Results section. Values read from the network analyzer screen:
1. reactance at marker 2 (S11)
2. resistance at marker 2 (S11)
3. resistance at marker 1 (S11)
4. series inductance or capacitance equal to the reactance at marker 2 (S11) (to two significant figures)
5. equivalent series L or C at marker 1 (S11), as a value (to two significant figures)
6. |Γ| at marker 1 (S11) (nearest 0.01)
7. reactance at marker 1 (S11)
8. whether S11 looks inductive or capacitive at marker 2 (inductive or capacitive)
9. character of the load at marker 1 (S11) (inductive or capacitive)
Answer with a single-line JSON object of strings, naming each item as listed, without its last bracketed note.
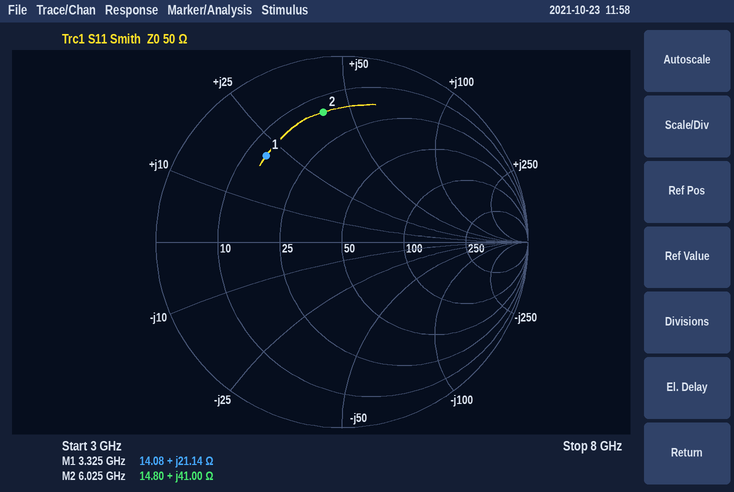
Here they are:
{"reactance at marker 2": "+41.00 Ω", "resistance at marker 2": "14.80 Ω", "resistance at marker 1": "14.08 Ω", "series inductance or capacitance equal to the reactance at marker 2 (S11)": "1.1 nH", "equivalent series L or C at marker 1 (S11), as a value": "1.0 nH", "|Γ| at marker 1 (S11)": "0.62", "reactance at marker 1": "+21.14 Ω", "whether S11 looks inductive or capacitive at marker 2": "inductive", "character of the load at marker 1 (S11)": "inductive"}
